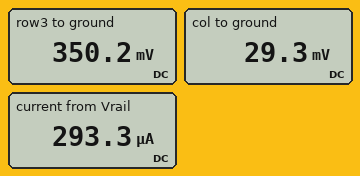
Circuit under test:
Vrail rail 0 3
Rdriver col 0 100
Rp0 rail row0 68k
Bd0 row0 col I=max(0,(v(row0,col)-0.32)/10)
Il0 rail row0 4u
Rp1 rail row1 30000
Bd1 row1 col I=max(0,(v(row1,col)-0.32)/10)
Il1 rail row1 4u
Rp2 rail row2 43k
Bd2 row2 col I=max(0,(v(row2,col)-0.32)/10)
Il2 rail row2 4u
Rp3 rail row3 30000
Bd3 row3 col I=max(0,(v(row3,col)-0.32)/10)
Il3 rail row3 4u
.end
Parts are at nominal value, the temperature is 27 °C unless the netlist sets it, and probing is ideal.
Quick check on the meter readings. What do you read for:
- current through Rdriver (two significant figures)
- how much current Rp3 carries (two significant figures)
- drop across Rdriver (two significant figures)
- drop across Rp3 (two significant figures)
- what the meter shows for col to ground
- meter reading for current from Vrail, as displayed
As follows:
290 µA
88 µA
29 mV
2.6 V
29.3 mV
293.3 µA
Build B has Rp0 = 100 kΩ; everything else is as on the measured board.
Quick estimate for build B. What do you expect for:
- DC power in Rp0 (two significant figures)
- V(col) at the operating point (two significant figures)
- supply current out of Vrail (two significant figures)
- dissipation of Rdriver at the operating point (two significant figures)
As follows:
70 µW
28 mV
280 µA
7.9 µW
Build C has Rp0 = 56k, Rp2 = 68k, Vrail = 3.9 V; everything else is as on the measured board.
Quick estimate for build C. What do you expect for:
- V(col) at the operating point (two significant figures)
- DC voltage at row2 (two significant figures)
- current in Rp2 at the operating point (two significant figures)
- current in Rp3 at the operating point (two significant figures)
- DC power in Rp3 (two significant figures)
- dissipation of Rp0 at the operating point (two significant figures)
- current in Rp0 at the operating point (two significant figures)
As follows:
37 mV
360 mV
52 µA
120 µA
420 µW
220 µW
63 µA
